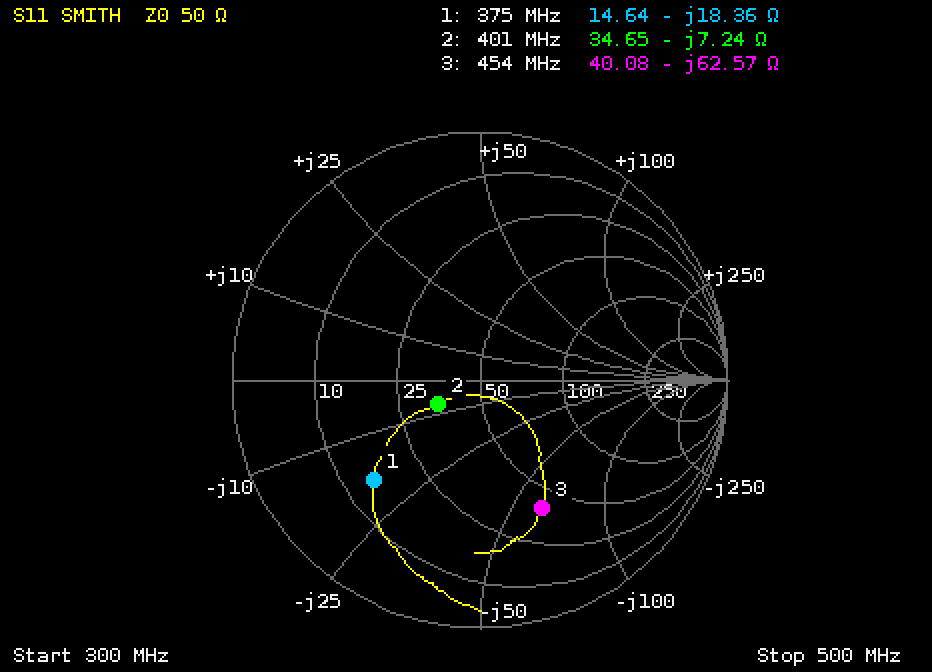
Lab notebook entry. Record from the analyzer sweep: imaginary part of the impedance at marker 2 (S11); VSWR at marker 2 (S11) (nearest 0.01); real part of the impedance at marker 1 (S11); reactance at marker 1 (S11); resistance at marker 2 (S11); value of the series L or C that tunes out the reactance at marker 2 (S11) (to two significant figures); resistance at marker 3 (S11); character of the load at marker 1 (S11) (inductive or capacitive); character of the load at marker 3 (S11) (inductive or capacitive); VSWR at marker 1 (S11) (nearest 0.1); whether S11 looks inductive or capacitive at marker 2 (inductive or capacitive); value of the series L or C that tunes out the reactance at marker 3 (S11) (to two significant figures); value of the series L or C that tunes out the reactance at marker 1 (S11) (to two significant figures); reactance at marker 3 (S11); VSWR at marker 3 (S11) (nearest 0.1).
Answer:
-7.24 Ω
1.50
14.64 Ω
-18.36 Ω
34.65 Ω
2.9 nH
40.08 Ω
capacitive
capacitive
3.9
capacitive
22 nH
7.8 nH
-62.57 Ω
3.7
